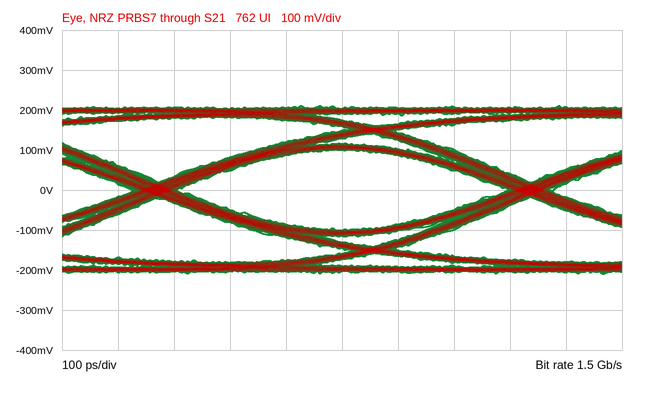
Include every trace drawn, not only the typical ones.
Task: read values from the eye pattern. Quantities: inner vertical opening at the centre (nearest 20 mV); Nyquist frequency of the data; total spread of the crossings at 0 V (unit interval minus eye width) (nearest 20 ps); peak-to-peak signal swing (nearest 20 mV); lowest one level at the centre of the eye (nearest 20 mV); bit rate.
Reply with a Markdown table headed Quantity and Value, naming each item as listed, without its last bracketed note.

| Quantity | Value |
|---|---|
| inner vertical opening at the centre | 200 mV |
| Nyquist frequency of the data | 750 MHz |
| total spread of the crossings at 0 V (unit interval minus eye width) | 80 ps |
| peak-to-peak signal swing | 420 mV |
| lowest one level at the centre of the eye | 100 mV |
| bit rate | 1.5 Gb/s |
